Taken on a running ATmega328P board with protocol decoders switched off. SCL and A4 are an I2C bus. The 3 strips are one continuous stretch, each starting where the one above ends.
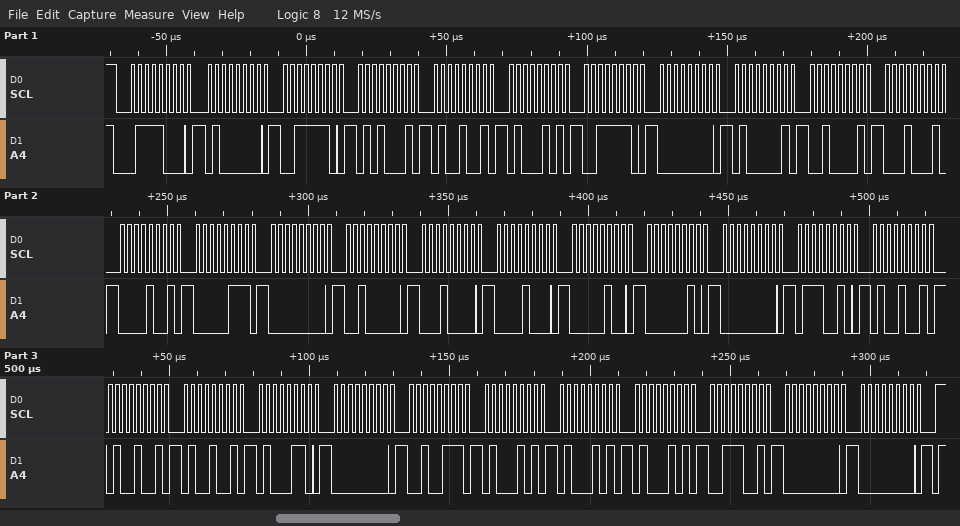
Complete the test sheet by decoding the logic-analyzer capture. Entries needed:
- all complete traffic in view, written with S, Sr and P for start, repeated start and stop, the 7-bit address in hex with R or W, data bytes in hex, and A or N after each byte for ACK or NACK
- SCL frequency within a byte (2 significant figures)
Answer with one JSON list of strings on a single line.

["S 3CW A 40 A 3E A 51 A 49 A 45 A 3E A 00 A 41 A 21 A 11 A 09 A 07 A 00 A 20 A 10 A 08 A 04 A 02 A 00 A 72 A 49 A 49 A 49 A 46 A 00 A 27 A 45 A 45 A 45 A 39 A 00 A 00 A P", "400 kHz"]
